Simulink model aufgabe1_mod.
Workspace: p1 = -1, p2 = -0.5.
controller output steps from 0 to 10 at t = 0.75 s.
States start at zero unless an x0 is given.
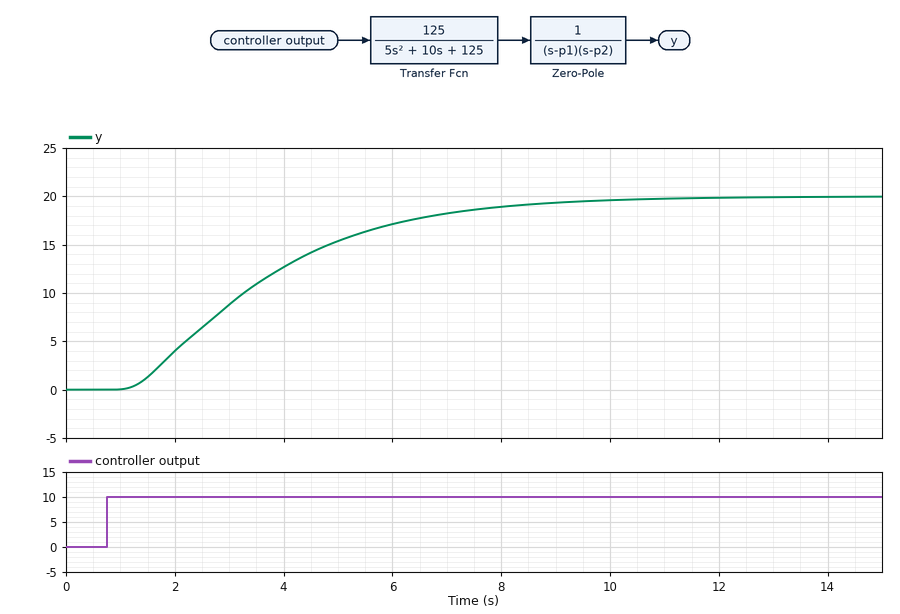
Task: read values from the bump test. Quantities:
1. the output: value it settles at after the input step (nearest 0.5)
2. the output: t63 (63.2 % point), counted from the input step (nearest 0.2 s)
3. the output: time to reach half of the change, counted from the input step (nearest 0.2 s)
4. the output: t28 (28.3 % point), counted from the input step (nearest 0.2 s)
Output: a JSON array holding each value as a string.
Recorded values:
["20.0", "3.2 s", "2.6 s", "1.6 s"]
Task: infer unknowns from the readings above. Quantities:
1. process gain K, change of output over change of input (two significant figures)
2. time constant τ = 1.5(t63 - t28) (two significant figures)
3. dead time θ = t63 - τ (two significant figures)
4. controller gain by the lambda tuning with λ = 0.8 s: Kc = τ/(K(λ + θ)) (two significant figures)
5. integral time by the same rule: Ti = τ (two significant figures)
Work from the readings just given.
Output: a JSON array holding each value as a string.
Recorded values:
["2.0", "2.4 s", "0.80 s", "0.75", "2.4 s"]
